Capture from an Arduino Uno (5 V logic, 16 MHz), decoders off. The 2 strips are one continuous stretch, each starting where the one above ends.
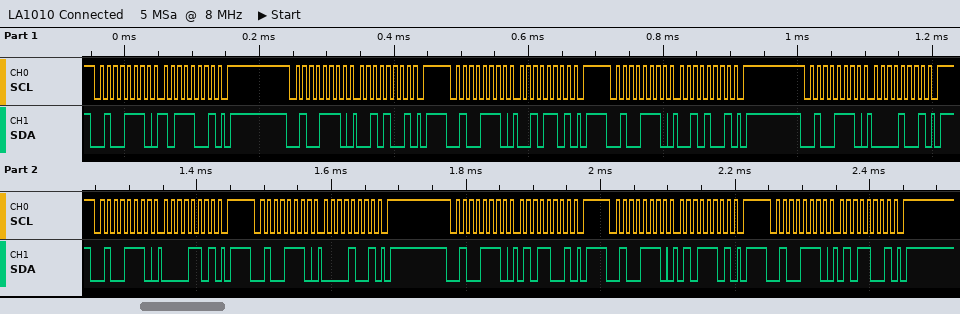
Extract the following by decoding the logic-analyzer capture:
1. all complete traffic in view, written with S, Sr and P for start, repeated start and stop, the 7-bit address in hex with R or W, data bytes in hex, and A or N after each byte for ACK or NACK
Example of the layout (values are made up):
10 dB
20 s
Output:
S 27W A B9 A P S 27W A 29 A P S 27W A 2D A P S 27W A 29 A P S 27W A 09 A P S 27W A 0D A P S 27W A 09 A P S 27W A 59 A P S 27W A 5D A P S 27W A 59 A P
